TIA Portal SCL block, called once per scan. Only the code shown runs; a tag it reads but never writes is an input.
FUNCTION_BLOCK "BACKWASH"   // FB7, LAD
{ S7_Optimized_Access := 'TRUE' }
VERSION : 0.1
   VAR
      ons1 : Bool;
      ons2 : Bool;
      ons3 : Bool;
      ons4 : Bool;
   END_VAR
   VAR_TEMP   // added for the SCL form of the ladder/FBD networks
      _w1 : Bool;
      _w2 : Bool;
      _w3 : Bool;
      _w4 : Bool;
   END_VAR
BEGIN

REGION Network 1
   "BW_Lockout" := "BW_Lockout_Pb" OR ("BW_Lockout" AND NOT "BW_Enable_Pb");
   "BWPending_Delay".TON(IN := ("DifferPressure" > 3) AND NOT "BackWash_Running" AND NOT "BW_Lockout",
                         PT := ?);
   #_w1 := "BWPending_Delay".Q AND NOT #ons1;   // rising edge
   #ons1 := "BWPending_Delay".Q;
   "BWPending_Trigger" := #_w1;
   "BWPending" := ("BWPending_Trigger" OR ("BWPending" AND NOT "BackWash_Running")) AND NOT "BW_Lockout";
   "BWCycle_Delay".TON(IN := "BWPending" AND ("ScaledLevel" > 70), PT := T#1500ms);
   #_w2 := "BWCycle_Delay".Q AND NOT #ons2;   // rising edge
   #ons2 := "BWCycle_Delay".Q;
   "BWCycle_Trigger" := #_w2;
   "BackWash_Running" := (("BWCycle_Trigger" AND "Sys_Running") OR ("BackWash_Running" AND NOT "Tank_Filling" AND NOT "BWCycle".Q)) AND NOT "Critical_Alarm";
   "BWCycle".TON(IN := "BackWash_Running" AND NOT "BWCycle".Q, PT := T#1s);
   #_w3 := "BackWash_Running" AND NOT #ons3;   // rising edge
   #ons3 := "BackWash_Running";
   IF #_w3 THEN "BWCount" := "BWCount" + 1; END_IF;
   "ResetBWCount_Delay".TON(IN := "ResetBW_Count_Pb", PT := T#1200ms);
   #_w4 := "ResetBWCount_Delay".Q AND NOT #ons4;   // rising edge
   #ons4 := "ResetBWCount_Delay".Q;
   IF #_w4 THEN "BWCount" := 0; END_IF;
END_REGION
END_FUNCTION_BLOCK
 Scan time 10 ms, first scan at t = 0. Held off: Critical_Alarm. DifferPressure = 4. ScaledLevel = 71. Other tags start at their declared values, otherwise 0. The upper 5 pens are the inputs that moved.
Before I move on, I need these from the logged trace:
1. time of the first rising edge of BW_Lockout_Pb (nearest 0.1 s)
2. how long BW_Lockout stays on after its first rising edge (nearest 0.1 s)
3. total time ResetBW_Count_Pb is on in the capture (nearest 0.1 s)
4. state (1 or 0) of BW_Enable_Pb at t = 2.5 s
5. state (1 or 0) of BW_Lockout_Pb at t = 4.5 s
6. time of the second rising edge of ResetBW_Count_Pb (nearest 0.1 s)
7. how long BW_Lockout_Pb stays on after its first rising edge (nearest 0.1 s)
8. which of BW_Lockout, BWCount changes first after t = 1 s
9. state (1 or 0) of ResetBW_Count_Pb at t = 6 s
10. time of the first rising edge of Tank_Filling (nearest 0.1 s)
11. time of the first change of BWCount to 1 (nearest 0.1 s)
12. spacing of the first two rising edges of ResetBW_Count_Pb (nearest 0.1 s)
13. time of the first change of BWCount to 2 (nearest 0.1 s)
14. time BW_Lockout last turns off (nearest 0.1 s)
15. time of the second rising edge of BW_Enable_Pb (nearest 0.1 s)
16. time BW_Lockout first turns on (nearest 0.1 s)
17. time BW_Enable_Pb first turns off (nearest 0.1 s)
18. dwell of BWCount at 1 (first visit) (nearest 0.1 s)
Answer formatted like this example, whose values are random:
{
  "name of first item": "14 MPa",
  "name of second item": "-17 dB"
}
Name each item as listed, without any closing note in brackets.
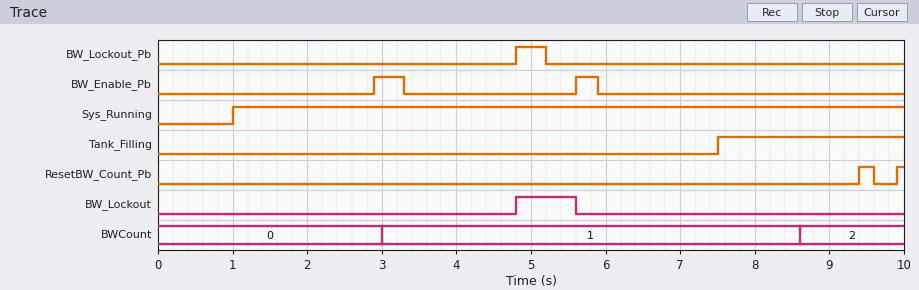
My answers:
{
  "time of the first rising edge of BW_Lockout_Pb": "4.8 s",
  "how long BW_Lockout stays on after its first rising edge": "0.8 s",
  "total time ResetBW_Count_Pb is on in the capture": "0.3 s",
  "state (1 or 0) of BW_Enable_Pb at t = 2.5 s": "0",
  "state (1 or 0) of BW_Lockout_Pb at t = 4.5 s": "0",
  "time of the second rising edge of ResetBW_Count_Pb": "9.9 s",
  "how long BW_Lockout_Pb stays on after its first rising edge": "0.4 s",
  "which of BW_Lockout, BWCount changes first after t = 1 s": "BWCount",
  "state (1 or 0) of ResetBW_Count_Pb at t = 6 s": "0",
  "time of the first rising edge of Tank_Filling": "7.5 s",
  "time of the first change of BWCount to 1": "3.0 s",
  "spacing of the first two rising edges of ResetBW_Count_Pb": "0.5 s",
  "time of the first change of BWCount to 2": "8.6 s",
  "time BW_Lockout last turns off": "5.6 s",
  "time of the second rising edge of BW_Enable_Pb": "5.6 s",
  "time BW_Lockout first turns on": "4.8 s",
  "time BW_Enable_Pb first turns off": "3.3 s",
  "dwell of BWCount at 1 (first visit)": "5.6 s"
}
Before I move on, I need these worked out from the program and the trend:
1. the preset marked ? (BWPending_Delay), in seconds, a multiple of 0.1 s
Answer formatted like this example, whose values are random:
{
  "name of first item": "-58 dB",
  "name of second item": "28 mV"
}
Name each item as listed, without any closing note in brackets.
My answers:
{
  "the preset marked ? (BWPending_Delay), in seconds, a multiple of 0.1 s": "1.5 s"
}
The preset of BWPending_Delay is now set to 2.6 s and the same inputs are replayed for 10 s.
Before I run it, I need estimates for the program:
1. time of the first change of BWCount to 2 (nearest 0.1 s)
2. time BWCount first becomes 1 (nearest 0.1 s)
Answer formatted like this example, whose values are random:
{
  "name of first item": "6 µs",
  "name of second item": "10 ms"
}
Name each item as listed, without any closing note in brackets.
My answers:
{
  "time of the first change of BWCount to 2": "9.7 s",
  "time BWCount first becomes 1": "4.1 s"
}
